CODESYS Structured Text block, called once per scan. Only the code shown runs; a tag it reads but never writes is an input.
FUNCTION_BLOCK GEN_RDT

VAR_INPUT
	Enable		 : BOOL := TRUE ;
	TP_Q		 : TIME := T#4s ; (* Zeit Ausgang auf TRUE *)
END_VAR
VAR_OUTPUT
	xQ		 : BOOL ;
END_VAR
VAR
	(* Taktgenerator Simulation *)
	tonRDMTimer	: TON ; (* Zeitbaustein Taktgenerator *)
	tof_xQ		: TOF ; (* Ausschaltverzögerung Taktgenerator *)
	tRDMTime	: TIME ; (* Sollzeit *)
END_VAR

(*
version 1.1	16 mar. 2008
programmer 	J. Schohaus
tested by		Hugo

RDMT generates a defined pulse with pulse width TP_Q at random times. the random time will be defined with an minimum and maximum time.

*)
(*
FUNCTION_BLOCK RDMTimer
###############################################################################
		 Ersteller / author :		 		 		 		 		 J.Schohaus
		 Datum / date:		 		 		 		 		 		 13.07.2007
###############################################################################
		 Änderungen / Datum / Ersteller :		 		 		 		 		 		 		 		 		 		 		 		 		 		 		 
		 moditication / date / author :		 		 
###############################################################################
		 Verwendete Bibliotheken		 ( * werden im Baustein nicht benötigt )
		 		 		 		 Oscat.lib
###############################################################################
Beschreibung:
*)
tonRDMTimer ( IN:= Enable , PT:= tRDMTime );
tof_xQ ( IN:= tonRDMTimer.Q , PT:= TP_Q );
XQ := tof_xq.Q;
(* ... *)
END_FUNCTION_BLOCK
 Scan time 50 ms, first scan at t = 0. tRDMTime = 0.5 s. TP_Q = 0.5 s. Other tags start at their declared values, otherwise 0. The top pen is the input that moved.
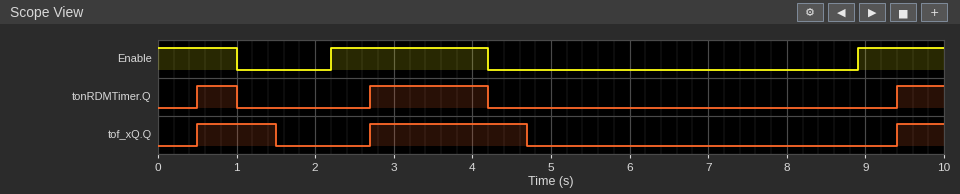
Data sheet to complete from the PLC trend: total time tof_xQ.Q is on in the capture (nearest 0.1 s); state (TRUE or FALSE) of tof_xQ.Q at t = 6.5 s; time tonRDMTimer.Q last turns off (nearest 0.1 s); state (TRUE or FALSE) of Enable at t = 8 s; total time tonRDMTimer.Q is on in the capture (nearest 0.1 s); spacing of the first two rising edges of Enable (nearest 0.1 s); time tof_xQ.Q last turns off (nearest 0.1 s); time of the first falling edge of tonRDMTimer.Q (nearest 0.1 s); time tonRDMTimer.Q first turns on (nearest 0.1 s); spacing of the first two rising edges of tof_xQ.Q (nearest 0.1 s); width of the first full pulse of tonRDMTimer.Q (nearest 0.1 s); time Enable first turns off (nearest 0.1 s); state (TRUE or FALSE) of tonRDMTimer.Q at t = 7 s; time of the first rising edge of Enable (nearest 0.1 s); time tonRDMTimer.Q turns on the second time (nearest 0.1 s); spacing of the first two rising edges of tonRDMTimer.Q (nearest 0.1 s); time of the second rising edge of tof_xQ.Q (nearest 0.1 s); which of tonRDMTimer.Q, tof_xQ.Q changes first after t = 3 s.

3.6 s
FALSE
4.2 s
FALSE
2.6 s
6.7 s
4.7 s
1.0 s
0.5 s
2.2 s
0.5 s
1.0 s
FALSE
2.2 s
2.7 s
2.2 s
2.7 s
tonRDMTimer.Q
